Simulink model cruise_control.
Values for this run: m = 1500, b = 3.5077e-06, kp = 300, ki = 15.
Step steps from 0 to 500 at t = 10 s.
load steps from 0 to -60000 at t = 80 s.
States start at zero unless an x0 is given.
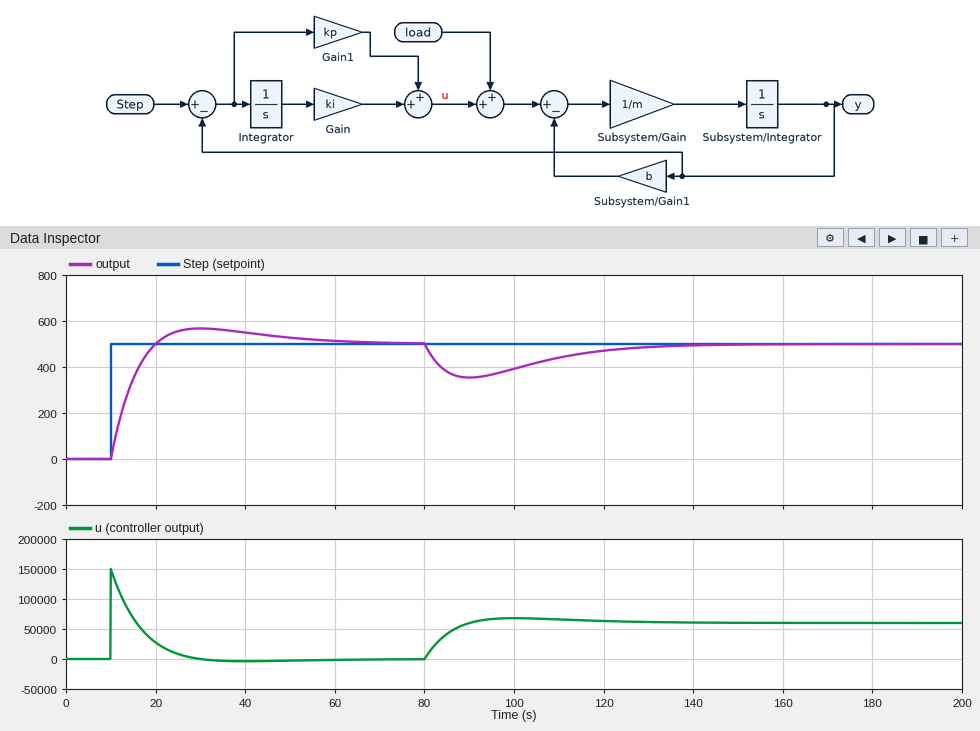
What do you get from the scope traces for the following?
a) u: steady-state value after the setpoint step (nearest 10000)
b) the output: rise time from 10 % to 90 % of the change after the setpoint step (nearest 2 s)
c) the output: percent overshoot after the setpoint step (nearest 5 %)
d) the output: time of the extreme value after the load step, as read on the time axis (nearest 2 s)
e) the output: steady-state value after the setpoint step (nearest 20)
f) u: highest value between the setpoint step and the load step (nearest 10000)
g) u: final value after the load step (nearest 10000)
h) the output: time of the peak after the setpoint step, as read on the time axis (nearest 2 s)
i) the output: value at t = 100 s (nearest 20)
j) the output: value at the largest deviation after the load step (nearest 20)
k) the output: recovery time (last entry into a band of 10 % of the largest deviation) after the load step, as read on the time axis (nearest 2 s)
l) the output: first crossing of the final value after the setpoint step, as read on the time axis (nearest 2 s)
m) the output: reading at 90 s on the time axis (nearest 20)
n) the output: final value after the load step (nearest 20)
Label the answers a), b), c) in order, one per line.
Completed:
a) 0
b) 8 s
c) 15 %
d) 90 s
e) 500
f) 150000
g) 60000
h) 30 s
i) 400
j) 360
k) 128 s
l) 20 s
m) 360
n) 500
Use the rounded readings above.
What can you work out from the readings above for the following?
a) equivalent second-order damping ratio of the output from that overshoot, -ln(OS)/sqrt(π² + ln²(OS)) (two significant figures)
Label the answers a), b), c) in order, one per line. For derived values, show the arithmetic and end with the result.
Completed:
a) ln(0.15) = -1.897; 1.897 / sqrt(9.870 + 3.599) = 0.52
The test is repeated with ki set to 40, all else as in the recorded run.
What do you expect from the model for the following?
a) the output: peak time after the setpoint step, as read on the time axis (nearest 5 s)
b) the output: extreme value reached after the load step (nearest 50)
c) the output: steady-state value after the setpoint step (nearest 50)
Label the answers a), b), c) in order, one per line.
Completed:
a) 25 s
b) 400
c) 500
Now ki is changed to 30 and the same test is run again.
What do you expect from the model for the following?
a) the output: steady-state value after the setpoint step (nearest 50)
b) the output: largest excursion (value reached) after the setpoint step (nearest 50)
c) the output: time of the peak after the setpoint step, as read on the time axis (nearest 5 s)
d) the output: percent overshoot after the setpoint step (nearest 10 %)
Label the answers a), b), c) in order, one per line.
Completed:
a) 500
b) 600
c) 25 s
d) 20 %
